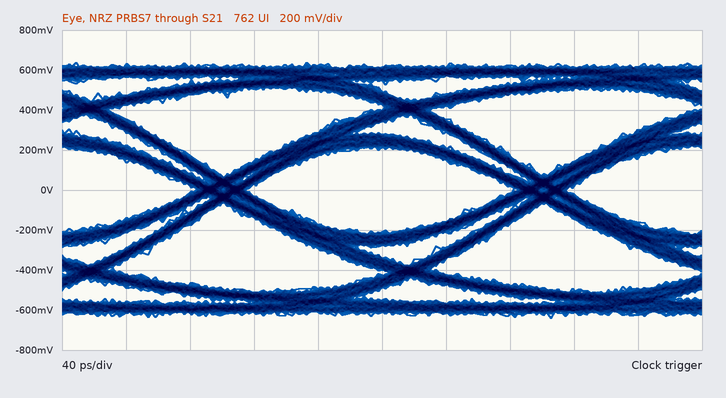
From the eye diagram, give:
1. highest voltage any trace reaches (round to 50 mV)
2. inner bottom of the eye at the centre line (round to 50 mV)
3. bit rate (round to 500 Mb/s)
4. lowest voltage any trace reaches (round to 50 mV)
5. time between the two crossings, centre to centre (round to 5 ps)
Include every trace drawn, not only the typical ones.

650 mV
-200 mV
5.0 Gb/s
-650 mV
200 ps
